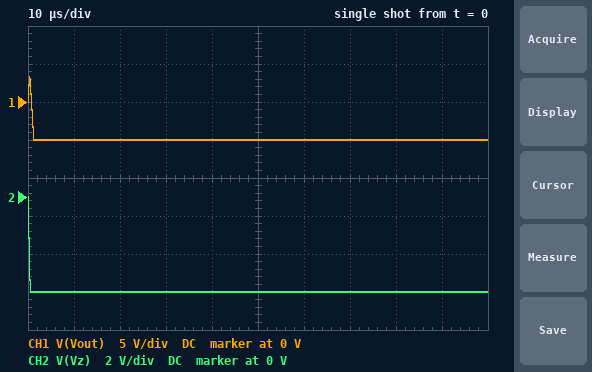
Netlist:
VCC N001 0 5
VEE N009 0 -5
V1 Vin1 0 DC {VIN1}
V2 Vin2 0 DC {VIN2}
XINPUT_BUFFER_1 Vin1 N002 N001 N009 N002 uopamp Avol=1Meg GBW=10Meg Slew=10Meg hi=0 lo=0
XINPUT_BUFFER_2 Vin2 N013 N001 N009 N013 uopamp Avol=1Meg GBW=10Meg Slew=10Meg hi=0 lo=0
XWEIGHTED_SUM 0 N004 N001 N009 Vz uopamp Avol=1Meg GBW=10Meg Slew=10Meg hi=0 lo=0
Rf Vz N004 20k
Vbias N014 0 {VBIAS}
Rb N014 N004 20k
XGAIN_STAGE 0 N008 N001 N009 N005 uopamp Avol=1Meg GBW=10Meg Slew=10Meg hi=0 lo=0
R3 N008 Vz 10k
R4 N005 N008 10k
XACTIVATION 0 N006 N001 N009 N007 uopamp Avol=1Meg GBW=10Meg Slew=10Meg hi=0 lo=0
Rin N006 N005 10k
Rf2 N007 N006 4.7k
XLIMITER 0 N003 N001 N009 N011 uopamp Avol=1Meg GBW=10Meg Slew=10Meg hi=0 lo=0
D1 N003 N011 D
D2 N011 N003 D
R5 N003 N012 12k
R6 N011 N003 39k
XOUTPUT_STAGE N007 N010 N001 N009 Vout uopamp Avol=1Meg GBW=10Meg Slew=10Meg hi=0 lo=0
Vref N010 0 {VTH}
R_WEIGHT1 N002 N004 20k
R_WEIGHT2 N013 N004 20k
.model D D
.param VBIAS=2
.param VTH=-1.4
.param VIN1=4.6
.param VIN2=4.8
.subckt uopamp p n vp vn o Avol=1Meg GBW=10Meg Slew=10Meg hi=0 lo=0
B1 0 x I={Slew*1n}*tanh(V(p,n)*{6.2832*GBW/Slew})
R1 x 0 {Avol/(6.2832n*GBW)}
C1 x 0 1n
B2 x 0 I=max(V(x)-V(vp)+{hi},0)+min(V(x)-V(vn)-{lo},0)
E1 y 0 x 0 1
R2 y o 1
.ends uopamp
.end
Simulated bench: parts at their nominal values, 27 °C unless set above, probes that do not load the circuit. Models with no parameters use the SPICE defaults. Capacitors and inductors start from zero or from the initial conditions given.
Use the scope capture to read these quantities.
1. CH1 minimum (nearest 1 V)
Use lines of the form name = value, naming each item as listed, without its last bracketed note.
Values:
CH1 minimum = -5 V
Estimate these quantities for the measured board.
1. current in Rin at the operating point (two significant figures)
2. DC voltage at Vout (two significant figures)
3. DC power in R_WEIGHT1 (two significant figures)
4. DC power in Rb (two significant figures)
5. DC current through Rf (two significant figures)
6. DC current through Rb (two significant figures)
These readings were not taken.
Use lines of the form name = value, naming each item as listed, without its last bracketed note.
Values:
current in Rin at the operating point = 500 µA
DC voltage at Vout = -5.0 V
DC power in R_WEIGHT1 = 450 µW
DC power in Rb = 8.1 µW
DC current through Rf = 330 µA
DC current through Rb = 20 µA
